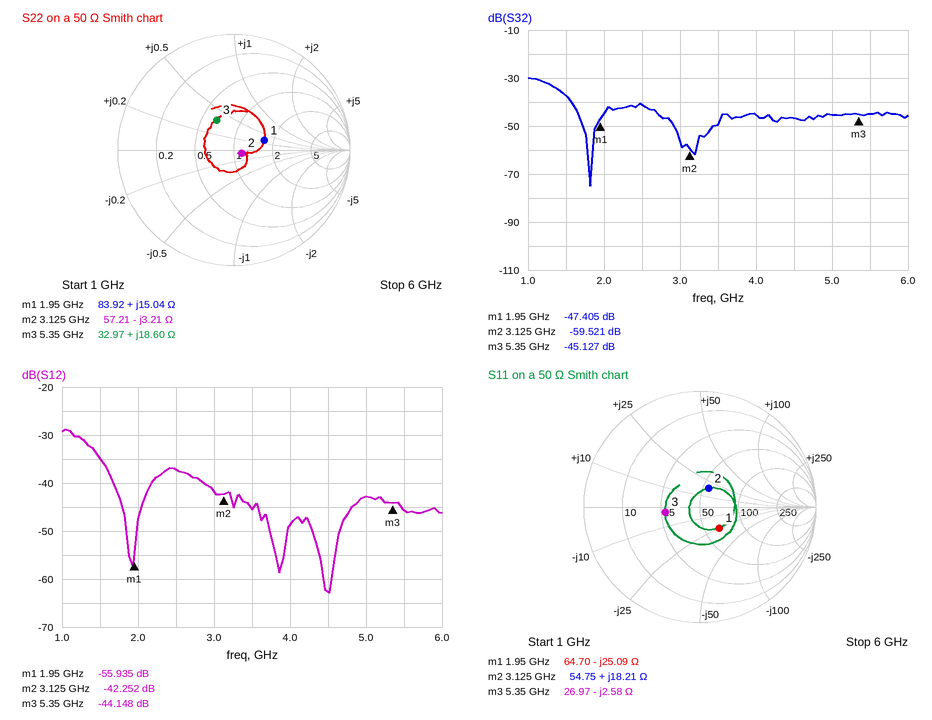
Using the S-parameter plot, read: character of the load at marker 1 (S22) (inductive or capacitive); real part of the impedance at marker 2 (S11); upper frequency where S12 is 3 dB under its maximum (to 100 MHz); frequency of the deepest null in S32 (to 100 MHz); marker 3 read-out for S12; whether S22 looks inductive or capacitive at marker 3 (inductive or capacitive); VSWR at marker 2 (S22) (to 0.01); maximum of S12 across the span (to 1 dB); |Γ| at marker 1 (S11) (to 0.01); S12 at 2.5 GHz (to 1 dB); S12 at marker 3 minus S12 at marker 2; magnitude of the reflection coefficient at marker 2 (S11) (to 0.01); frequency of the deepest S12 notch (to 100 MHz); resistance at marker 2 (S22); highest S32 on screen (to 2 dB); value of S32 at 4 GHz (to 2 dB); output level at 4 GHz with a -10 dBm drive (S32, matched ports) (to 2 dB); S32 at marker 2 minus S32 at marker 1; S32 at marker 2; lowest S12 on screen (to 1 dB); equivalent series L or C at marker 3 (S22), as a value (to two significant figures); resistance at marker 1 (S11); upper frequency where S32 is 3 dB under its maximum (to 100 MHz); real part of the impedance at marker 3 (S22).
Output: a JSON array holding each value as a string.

["inductive", "54.75 Ω", "1.3 GHz", "1.8 GHz", "-44.148 dB", "inductive", "1.16", "-29 dB", "0.25", "-37 dB", "-1.896 dB", "0.18", "4.5 GHz", "57.21 Ω", "-30 dB", "-46 dB", "-56 dBm", "-12.116 dB", "-59.521 dB", "-63 dB", "550 pH", "64.70 Ω", "1.3 GHz", "32.97 Ω"]
